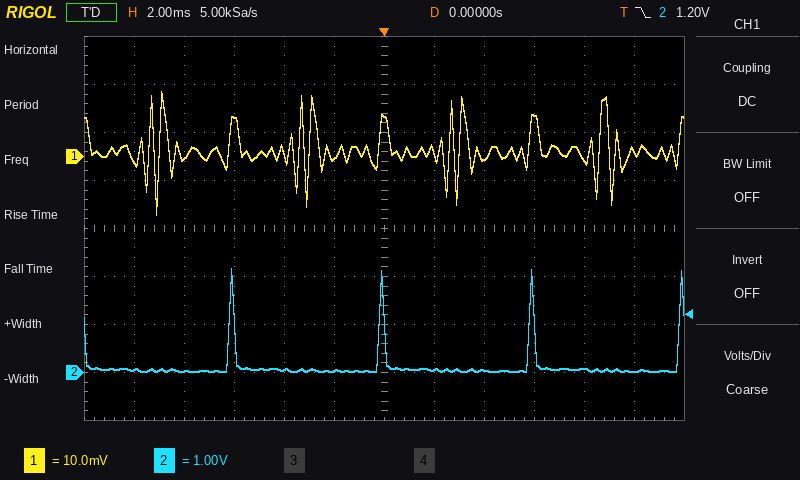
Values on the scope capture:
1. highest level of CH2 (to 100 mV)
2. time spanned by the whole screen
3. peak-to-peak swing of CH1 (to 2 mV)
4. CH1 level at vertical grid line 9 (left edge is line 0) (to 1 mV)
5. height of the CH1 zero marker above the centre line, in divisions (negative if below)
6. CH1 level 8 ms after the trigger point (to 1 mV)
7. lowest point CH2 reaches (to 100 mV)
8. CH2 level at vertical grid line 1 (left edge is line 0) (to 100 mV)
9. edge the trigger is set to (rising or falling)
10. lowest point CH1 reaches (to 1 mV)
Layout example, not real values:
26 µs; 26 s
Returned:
2.2 V; 24 ms; 26 mV; 8 mV; +1.5 div; -1 mV; 0.0 V; 100 mV; falling; -12 mV
